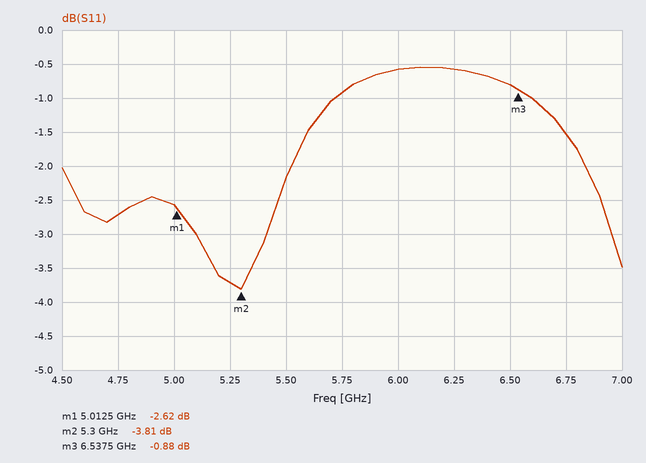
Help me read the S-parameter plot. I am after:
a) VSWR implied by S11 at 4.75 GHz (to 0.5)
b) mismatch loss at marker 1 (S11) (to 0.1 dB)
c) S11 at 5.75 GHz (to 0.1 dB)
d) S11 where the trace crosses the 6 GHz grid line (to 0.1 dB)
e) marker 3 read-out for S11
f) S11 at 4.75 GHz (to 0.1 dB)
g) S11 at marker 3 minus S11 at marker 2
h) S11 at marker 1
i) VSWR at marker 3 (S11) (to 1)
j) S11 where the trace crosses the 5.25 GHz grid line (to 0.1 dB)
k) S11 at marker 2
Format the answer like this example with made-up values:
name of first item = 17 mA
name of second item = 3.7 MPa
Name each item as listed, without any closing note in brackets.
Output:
VSWR implied by S11 at 4.75 GHz = 6.5
mismatch loss at marker 1 (S11) = 3.4 dB
S11 at 5.75 GHz = -0.9 dB
S11 where the trace crosses the 6 GHz grid line = -0.6 dB
marker 3 read-out for S11 = -0.88 dB
S11 at 4.75 GHz = -2.7 dB
S11 at marker 3 minus S11 at marker 2 = 2.93 dB
S11 at marker 1 = -2.62 dB
VSWR at marker 3 (S11) = 20
S11 where the trace crosses the 5.25 GHz grid line = -3.7 dB
S11 at marker 2 = -3.81 dB
